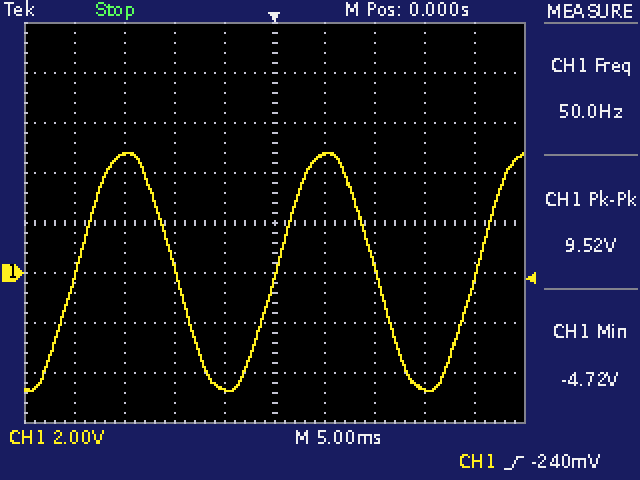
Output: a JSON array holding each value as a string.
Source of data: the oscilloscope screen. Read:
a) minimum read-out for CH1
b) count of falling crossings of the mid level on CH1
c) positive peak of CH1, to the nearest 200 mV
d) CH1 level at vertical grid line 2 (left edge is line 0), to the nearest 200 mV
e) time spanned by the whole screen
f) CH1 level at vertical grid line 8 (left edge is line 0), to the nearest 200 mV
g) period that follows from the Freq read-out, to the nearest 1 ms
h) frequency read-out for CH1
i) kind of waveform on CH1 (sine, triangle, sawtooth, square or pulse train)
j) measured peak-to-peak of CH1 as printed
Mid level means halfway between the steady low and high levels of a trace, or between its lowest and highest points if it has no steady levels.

["-4.72 V", "2", "4.8 V", "4.8 V", "50 ms", "-4.6 V", "20 ms", "50.0 Hz", "sine", "9.52 V"]
